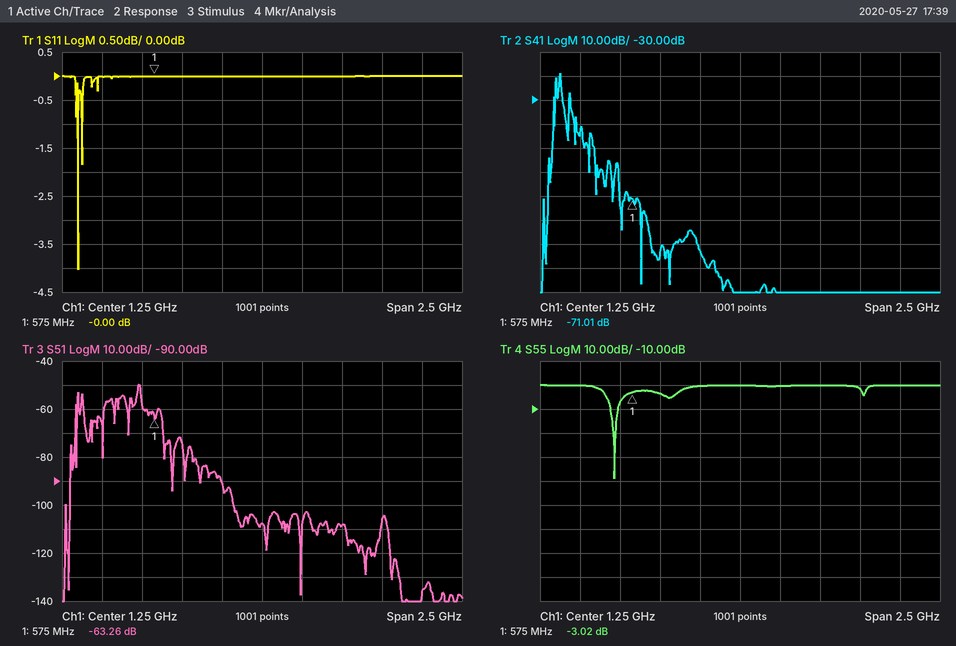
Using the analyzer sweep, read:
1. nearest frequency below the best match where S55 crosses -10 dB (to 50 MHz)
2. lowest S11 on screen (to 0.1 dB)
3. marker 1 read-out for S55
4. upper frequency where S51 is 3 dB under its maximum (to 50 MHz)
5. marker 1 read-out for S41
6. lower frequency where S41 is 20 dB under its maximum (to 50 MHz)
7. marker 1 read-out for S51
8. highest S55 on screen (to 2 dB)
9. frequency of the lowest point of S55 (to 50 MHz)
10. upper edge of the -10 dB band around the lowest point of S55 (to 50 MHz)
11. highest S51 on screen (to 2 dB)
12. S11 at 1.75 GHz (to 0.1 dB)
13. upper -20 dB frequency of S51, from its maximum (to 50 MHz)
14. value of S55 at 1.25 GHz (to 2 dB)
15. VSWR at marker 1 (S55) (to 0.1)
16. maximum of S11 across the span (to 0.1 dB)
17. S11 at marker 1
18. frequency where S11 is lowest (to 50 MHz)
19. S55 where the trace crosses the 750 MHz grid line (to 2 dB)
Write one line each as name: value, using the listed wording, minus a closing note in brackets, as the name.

nearest frequency below the best match where S55 crosses -10 dB: 450 MHz
lowest S11 on screen: -4.0 dB
marker 1 read-out for S55: -3.02 dB
upper frequency where S51 is 3 dB under its maximum: 500 MHz
marker 1 read-out for S41: -71.01 dB
lower frequency where S41 is 20 dB under its maximum: 100 MHz
marker 1 read-out for S51: -63.26 dB
highest S55 on screen: 0 dB
frequency of the lowest point of S55: 450 MHz
upper edge of the -10 dB band around the lowest point of S55: 500 MHz
highest S51 on screen: -50 dB
S11 at 1.75 GHz: 0.0 dB
upper -20 dB frequency of S51, from its maximum: 650 MHz
value of S55 at 1.25 GHz: 0 dB
VSWR at marker 1 (S55): 5.8
maximum of S11 across the span: 0.0 dB
S11 at marker 1: -0.00 dB
frequency where S11 is lowest: 100 MHz
S55 where the trace crosses the 750 MHz grid line: -4 dB
